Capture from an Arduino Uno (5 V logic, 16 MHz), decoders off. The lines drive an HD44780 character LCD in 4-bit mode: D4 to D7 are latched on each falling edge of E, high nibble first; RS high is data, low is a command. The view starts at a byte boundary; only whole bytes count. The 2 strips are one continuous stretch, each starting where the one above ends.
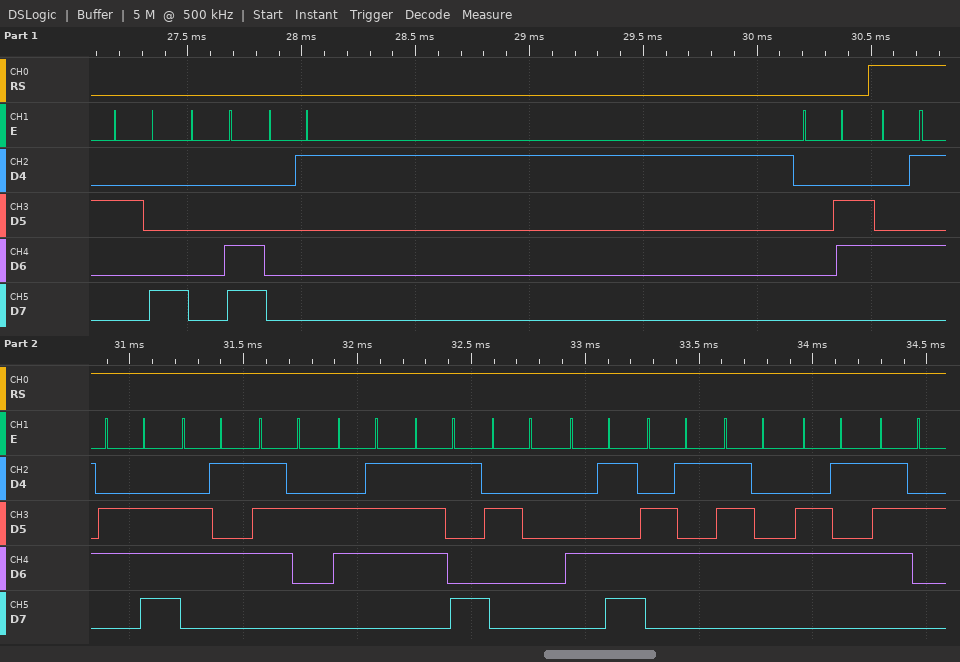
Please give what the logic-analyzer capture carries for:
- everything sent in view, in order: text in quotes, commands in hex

0x28 0x0C 0x01 0x06 "Energy Meter"
